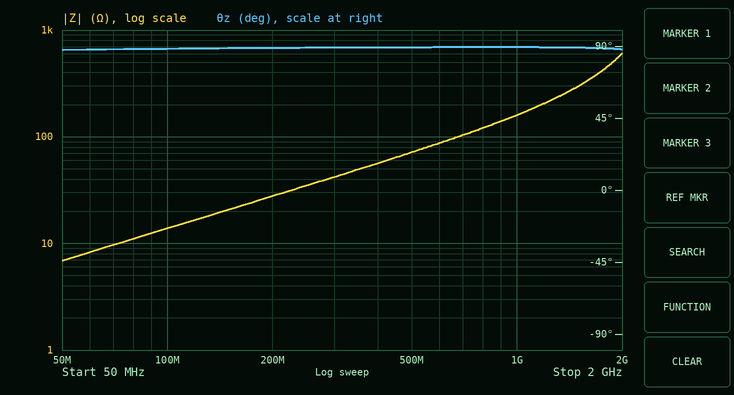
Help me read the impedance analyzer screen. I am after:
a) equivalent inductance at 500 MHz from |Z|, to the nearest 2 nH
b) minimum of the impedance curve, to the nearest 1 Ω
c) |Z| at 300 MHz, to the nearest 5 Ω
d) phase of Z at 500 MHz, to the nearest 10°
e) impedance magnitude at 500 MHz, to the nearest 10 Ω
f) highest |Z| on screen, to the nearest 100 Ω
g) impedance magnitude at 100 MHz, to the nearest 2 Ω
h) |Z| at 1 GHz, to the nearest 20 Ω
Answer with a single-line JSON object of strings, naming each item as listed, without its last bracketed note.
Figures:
{"equivalent inductance at 500 MHz from |Z|, to the nearest 2 nH": "22 nH", "minimum of the impedance curve, to the nearest 1 Ω": "7 Ω", "|Z| at 300 MHz, to the nearest 5 Ω": "40 Ω", "phase of Z at 500 MHz, to the nearest 10°": "90°", "impedance magnitude at 500 MHz, to the nearest 10 Ω": "70 Ω", "highest |Z| on screen, to the nearest 100 Ω": "600 Ω", "impedance magnitude at 100 MHz, to the nearest 2 Ω": "14 Ω", "|Z| at 1 GHz, to the nearest 20 Ω": "160 Ω"}
